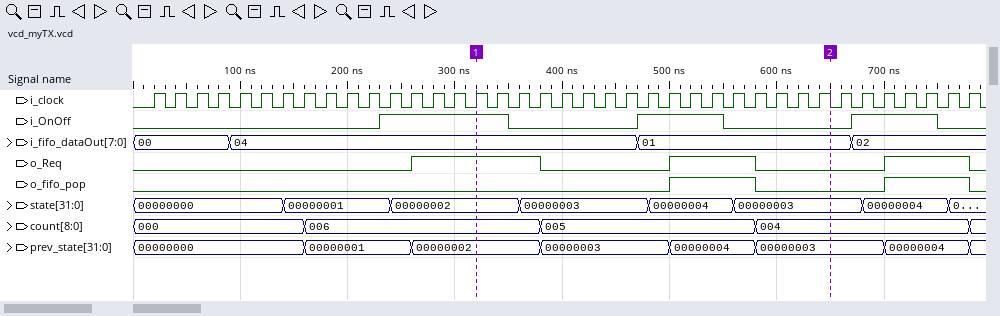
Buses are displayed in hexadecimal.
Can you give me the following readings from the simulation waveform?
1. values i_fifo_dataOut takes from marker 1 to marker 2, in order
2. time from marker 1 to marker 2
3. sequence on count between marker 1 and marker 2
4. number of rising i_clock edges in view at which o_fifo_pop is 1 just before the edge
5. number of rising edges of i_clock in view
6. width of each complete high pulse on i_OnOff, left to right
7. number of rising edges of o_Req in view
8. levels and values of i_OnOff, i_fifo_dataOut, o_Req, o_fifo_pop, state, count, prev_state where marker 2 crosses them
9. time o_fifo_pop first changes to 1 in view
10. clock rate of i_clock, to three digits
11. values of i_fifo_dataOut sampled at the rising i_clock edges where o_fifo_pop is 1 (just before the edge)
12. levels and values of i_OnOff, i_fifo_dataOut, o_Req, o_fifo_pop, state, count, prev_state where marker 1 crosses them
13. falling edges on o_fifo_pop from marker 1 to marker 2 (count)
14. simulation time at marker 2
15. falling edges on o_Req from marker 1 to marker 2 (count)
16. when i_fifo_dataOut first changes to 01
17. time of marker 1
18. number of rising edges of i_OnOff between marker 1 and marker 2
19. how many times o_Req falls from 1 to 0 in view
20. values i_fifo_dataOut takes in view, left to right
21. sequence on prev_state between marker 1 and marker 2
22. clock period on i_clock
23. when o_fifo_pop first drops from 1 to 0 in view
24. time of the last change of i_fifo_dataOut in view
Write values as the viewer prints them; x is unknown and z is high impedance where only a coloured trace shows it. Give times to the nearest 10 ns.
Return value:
04, 01
330 ns
006, 005, 004
8
39
120 ns, 80 ns, 80 ns
3
i_OnOff=0, i_fifo_dataOut=01, o_Req=0, o_fifo_pop=0, state=00000003, count=004, prev_state=00000003
500 ns
50.0 MHz
01, 01, 01, 01, 02, 02, 02, 02
i_OnOff=1, i_fifo_dataOut=04, o_Req=1, o_fifo_pop=0, state=00000002, count=006, prev_state=00000002
1
650 ns
2
470 ns
320 ns
1
3
00, 04, 01, 02
00000002, 00000003, 00000004, 00000003
20 ns
580 ns
670 ns
